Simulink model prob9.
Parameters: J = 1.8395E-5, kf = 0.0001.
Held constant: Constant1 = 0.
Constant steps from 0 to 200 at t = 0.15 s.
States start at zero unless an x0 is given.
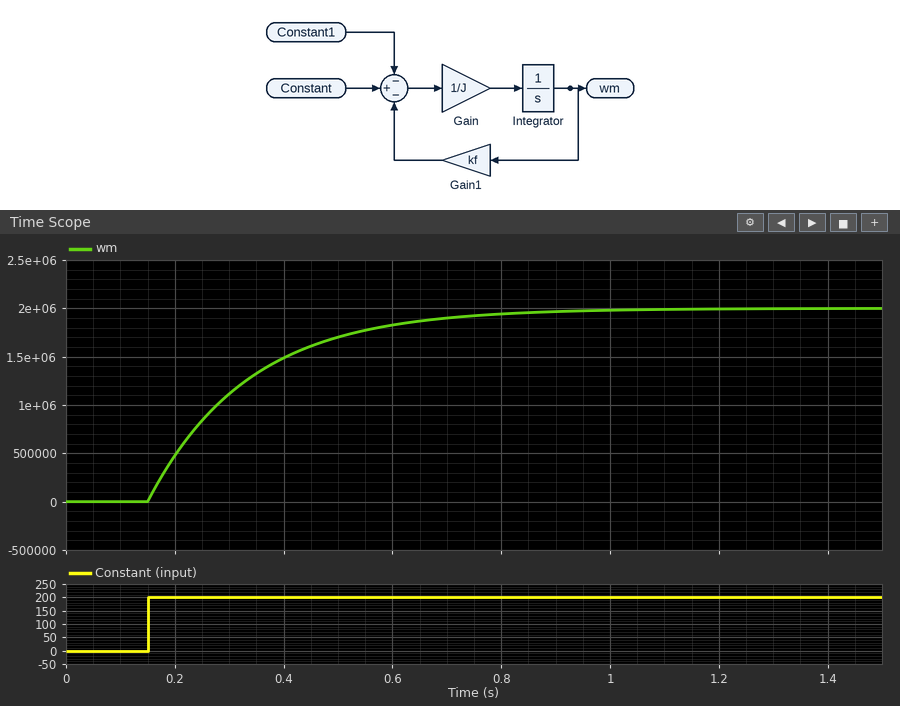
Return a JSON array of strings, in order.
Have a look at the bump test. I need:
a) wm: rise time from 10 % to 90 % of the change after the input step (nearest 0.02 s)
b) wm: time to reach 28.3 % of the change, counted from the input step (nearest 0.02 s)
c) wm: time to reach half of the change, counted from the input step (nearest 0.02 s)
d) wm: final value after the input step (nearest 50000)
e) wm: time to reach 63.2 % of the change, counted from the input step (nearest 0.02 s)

["0.40 s", "0.06 s", "0.12 s", "2000000", "0.18 s"]
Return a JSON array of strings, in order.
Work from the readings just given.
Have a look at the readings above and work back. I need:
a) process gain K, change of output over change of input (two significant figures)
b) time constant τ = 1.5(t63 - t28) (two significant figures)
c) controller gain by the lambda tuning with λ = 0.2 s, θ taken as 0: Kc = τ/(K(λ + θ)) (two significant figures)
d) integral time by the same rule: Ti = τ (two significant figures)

["10000", "0.18 s", "0.000090", "0.18 s"]
